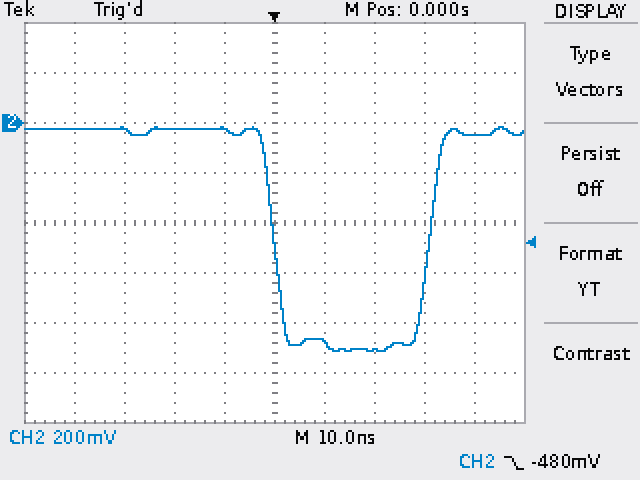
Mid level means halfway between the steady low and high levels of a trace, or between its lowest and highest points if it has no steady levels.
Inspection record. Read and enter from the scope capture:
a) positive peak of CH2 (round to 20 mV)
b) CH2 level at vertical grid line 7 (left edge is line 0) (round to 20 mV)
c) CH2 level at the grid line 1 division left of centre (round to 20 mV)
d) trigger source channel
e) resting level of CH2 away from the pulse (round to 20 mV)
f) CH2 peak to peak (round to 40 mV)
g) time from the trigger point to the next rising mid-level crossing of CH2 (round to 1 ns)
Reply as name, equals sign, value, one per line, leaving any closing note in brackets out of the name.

positive peak of CH2 = -20 mV
CH2 level at vertical grid line 7 (left edge is line 0) = -900 mV
CH2 level at the grid line 1 division left of centre = -20 mV
trigger source channel = CH2
resting level of CH2 away from the pulse = -20 mV
CH2 peak to peak = 880 mV
time from the trigger point to the next rising mid-level crossing of CH2 = 31 ns
